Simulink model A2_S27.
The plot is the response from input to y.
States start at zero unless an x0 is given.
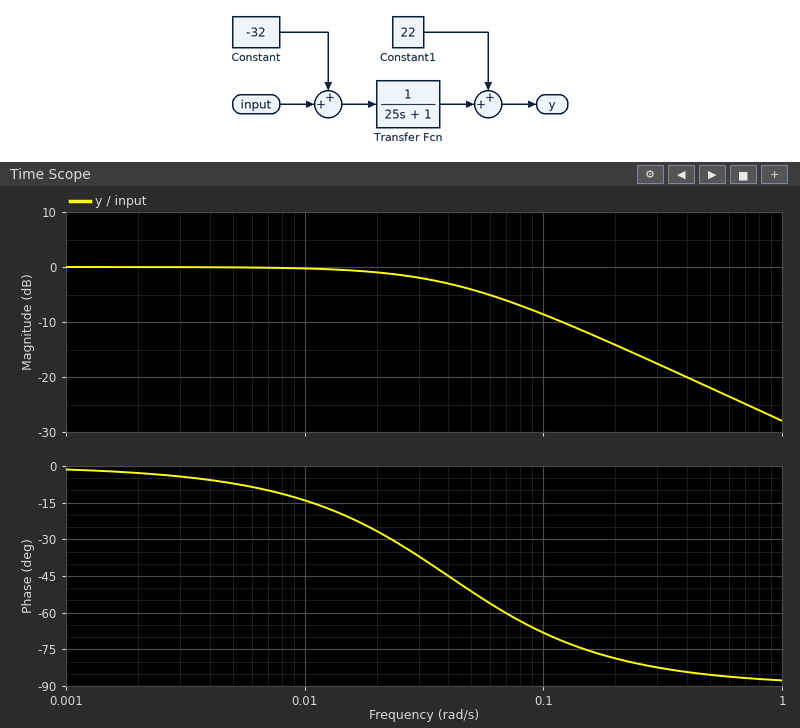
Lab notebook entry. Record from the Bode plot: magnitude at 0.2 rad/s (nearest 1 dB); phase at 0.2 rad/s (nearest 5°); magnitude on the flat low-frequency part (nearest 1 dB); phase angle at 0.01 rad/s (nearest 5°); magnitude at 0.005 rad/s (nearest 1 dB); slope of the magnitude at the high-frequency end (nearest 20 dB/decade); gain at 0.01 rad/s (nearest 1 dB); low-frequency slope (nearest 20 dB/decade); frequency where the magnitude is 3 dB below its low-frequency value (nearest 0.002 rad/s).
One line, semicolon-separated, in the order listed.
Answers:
-14 dB; -80°; 0 dB; -15°; 0 dB; -20 dB/decade; 0 dB; 0 dB/decade; 0.040 rad/s
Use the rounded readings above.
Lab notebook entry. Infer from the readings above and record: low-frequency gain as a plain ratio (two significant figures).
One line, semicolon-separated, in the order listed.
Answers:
1.0
